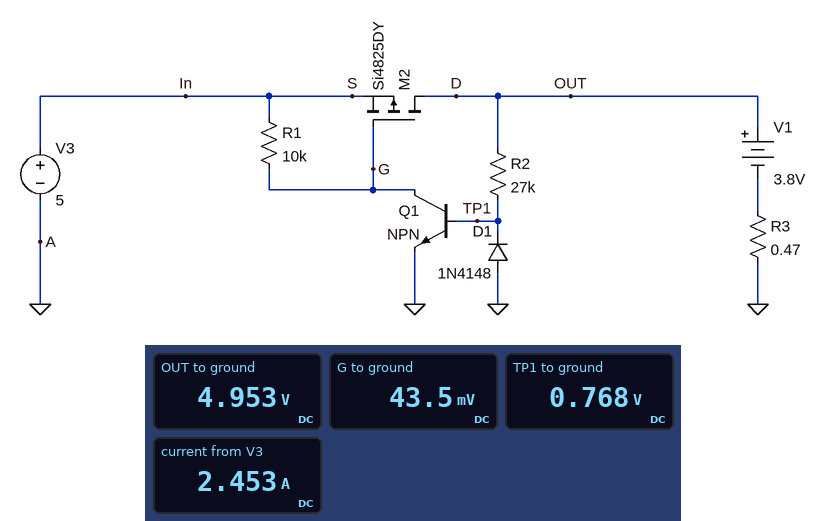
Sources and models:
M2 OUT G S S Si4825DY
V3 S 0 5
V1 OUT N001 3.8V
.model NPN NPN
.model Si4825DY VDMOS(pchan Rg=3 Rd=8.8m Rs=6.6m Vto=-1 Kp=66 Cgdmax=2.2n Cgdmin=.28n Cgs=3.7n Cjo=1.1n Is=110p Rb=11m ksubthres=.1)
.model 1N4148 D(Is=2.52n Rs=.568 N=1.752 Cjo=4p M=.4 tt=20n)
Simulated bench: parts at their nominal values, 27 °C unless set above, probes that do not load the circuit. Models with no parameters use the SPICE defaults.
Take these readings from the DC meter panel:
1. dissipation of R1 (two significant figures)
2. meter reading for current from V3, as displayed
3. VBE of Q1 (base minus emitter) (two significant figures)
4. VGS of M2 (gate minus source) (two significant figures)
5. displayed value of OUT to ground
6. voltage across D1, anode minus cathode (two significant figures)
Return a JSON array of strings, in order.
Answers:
["2.5 mW", "2.453 A", "770 mV", "-5.0 V", "4.953 V", "-770 mV"]
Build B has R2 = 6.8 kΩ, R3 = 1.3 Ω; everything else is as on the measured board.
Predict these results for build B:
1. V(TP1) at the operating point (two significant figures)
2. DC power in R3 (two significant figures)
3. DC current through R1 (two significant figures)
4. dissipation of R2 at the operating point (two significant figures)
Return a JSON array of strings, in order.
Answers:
["790 mV", "1.1 W", "500 µA", "2.6 mW"]
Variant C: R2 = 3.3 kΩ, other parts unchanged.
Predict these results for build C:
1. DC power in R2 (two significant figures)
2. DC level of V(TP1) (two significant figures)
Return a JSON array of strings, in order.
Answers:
["5.2 mW", "800 mV"]
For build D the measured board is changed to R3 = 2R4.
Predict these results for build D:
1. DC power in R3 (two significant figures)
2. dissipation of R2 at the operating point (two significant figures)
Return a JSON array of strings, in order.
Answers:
["590 mW", "660 µW"]
